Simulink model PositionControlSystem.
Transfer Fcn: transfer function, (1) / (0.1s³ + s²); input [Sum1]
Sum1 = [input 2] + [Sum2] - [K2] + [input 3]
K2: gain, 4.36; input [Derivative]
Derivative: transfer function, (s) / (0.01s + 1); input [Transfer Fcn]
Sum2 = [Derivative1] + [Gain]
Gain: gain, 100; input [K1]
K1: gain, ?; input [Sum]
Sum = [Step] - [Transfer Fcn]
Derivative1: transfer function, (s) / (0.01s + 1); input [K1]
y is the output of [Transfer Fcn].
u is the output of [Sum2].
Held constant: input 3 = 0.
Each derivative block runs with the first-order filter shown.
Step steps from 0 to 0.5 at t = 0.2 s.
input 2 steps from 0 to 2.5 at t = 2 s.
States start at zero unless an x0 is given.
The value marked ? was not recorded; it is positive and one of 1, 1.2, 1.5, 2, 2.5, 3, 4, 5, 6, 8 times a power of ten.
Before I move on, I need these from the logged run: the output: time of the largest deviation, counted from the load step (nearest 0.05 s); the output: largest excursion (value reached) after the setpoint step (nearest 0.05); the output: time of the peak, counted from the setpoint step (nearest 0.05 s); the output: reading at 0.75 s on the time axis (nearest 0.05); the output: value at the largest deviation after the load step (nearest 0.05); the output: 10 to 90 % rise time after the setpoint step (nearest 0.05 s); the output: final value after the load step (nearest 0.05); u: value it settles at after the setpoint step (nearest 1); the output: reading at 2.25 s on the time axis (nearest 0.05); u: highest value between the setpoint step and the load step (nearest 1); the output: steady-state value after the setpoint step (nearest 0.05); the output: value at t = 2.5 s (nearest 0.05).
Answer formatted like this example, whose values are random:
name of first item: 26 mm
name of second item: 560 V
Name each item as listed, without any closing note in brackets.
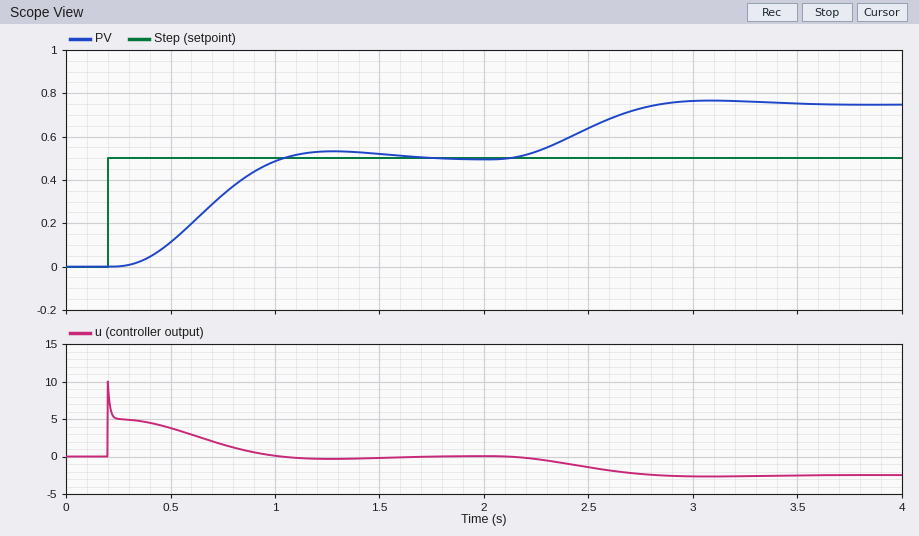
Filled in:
the output: time of the largest deviation, counted from the load step: 1.10 s
the output: largest excursion (value reached) after the setpoint step: 0.55
the output: time of the peak, counted from the setpoint step: 1.10 s
the output: reading at 0.75 s on the time axis: 0.35
the output: value at the largest deviation after the load step: 0.75
the output: 10 to 90 % rise time after the setpoint step: 0.50 s
the output: final value after the load step: 0.75
u: value it settles at after the setpoint step: 0
the output: reading at 2.25 s on the time axis: 0.55
u: highest value between the setpoint step and the load step: 10
the output: steady-state value after the setpoint step: 0.50
the output: value at t = 2.5 s: 0.65
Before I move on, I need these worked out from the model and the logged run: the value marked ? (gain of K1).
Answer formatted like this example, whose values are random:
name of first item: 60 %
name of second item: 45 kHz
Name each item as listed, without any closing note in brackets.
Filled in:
the value marked ?: 0.1
